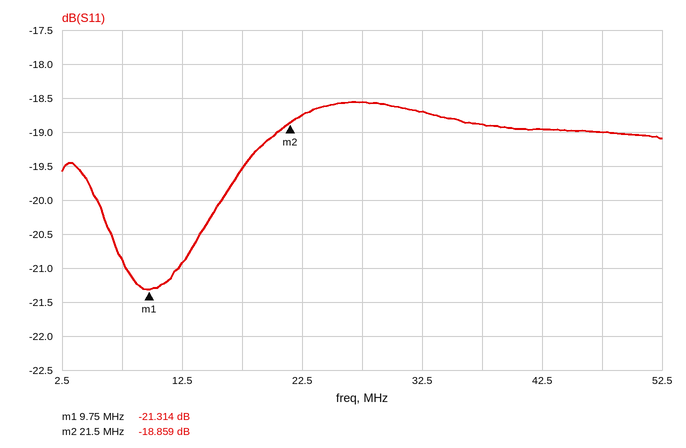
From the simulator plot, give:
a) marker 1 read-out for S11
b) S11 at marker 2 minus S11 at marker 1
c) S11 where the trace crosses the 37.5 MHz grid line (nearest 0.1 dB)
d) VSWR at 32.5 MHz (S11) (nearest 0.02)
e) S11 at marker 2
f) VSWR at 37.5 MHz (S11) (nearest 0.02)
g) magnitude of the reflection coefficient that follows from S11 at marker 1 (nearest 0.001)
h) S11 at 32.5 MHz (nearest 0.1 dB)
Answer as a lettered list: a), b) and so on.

a) -21.314 dB
b) 2.455 dB
c) -18.9 dB
d) 1.26
e) -18.859 dB
f) 1.26
g) 0.086
h) -18.7 dB
